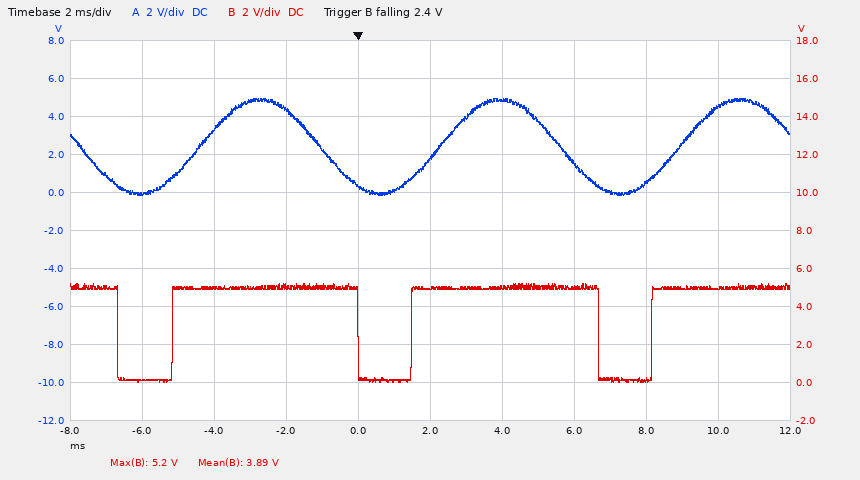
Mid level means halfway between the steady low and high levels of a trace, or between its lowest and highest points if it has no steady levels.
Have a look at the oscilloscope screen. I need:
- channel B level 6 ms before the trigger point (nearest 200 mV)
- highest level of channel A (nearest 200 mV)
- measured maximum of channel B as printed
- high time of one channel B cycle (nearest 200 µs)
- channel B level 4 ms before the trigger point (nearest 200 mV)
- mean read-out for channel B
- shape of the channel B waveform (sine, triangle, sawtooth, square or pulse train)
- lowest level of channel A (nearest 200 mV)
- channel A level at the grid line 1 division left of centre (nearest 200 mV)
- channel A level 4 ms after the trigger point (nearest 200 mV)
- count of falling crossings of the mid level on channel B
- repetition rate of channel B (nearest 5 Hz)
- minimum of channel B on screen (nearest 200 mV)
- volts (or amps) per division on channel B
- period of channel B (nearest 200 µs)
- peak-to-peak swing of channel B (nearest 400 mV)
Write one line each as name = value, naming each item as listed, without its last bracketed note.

channel B level 6 ms before the trigger point = 200 mV
highest level of channel A = 5.0 V
measured maximum of channel B as printed = 5.2 V
high time of one channel B cycle = 5.2 ms
channel B level 4 ms before the trigger point = 5.0 V
mean read-out for channel B = 3.89 V
shape of the channel B waveform = pulse train
lowest level of channel A = -200 mV
channel A level at the grid line 1 division left of centre = 400 mV
channel A level 4 ms after the trigger point = 4.8 V
count of falling crossings of the mid level on channel B = 3
repetition rate of channel B = 150 Hz
minimum of channel B on screen = 0.0 V
volts (or amps) per division on channel B = 2 V
period of channel B = 6.6 ms
peak-to-peak swing of channel B = 5.2 V
